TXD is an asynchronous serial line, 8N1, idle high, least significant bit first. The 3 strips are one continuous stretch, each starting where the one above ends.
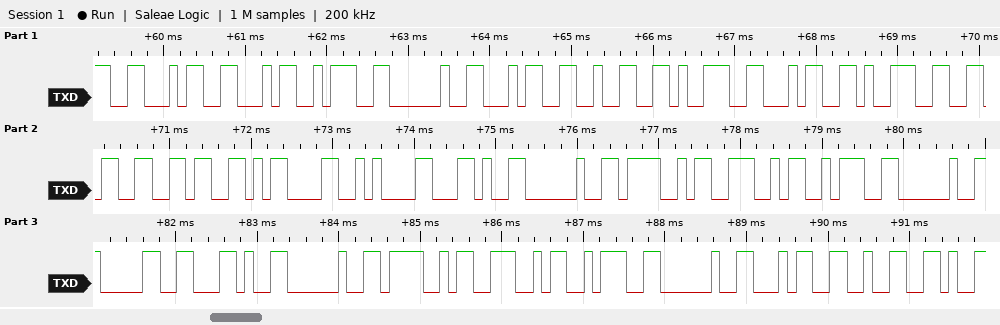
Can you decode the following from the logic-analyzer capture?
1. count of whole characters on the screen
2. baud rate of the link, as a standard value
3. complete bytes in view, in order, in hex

28
9600 baud
46 46 3A 20 34 32 39 34 39 36 36 0D 0A 2C 20 4F 4E 3A 20 30 2C 20 4F 4E 3A 20 34 32
